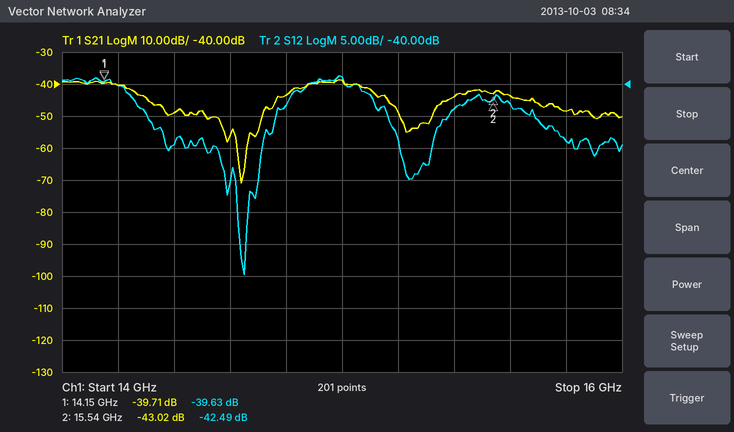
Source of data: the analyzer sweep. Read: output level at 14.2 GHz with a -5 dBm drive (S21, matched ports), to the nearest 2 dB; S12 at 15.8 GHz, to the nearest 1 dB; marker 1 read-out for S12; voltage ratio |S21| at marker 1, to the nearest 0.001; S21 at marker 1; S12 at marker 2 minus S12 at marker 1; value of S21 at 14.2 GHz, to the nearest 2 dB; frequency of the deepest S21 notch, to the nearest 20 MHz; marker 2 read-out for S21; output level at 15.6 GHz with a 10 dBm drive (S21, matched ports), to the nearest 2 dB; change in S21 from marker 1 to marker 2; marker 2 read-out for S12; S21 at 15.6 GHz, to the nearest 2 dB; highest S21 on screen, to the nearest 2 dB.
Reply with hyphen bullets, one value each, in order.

- -46 dBm
- -49 dB
- -39.63 dB
- 0.010
- -39.71 dB
- -2.86 dB
- -40 dB
- 14.64 GHz
- -43.02 dB
- -34 dBm
- -3.31 dB
- -42.49 dB
- -44 dB
- -38 dB
